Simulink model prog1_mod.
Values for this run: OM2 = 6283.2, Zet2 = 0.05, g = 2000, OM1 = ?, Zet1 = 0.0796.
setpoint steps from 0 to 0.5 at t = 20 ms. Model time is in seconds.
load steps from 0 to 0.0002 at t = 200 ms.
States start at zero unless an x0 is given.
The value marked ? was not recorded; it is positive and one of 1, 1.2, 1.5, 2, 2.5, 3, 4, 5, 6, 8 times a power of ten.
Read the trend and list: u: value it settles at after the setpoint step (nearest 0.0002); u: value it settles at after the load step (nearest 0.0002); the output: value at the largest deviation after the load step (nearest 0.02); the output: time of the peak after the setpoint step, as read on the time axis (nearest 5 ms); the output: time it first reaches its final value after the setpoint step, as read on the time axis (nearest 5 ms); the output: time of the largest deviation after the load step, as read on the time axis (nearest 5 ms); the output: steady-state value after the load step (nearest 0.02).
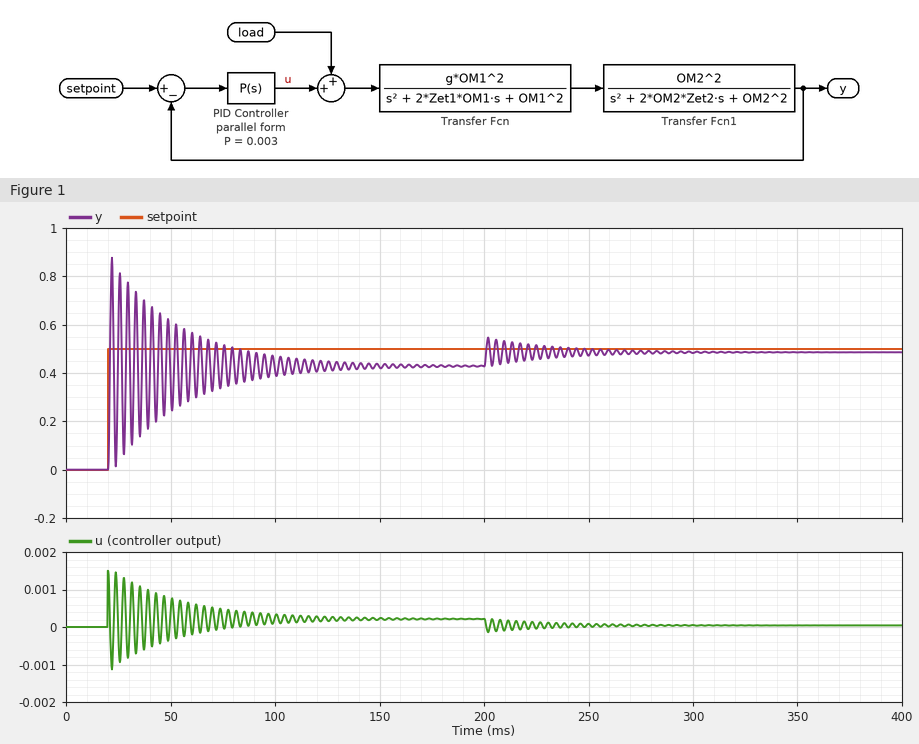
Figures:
0.0002
0.0000
0.54
20 ms
20 ms
200 ms
0.48
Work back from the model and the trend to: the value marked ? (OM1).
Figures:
600
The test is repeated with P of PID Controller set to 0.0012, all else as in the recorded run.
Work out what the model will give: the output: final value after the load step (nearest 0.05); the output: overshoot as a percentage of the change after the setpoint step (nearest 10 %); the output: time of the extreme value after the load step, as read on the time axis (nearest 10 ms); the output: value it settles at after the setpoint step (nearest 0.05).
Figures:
0.45
90 %
200 ms
0.35
